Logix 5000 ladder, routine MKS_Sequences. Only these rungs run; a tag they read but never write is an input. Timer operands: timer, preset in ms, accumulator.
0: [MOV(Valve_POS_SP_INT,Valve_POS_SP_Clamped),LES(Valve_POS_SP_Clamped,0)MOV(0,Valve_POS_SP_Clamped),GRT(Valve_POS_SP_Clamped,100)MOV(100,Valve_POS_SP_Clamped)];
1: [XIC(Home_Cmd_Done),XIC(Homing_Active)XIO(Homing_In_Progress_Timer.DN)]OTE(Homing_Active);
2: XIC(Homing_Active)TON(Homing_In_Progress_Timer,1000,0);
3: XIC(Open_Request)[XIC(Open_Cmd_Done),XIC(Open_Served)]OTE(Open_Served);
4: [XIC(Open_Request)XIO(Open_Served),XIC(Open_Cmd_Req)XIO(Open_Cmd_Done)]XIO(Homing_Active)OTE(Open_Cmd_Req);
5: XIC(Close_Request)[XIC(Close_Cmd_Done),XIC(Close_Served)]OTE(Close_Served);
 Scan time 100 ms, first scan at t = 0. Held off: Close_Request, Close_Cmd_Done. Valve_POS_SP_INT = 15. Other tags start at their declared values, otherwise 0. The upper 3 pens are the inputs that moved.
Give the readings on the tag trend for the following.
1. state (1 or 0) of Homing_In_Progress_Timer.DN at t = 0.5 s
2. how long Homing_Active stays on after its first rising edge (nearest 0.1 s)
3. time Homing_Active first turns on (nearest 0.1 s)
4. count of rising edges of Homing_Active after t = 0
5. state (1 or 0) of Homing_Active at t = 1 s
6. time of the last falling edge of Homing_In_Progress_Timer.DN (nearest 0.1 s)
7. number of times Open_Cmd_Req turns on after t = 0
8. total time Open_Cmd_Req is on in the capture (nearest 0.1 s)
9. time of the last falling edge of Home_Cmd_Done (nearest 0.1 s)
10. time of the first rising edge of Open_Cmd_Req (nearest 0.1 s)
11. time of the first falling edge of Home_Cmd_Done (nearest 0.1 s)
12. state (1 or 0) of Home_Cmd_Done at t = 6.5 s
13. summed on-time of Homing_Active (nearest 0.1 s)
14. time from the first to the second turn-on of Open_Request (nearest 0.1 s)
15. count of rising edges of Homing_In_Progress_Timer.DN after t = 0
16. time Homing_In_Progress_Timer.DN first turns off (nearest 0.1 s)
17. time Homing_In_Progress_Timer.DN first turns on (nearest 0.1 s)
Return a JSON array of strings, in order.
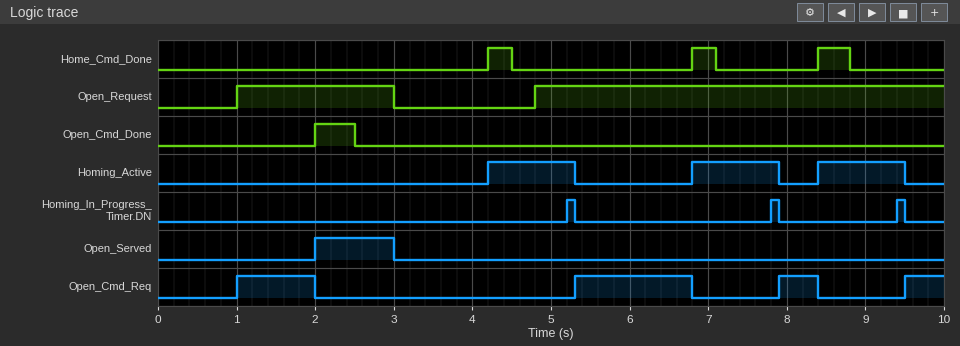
["0", "1.1 s", "4.2 s", "3", "0", "9.5 s", "4", "3.5 s", "8.8 s", "1.0 s", "4.5 s", "0", "3.3 s", "3.8 s", "3", "5.3 s", "5.2 s"]
